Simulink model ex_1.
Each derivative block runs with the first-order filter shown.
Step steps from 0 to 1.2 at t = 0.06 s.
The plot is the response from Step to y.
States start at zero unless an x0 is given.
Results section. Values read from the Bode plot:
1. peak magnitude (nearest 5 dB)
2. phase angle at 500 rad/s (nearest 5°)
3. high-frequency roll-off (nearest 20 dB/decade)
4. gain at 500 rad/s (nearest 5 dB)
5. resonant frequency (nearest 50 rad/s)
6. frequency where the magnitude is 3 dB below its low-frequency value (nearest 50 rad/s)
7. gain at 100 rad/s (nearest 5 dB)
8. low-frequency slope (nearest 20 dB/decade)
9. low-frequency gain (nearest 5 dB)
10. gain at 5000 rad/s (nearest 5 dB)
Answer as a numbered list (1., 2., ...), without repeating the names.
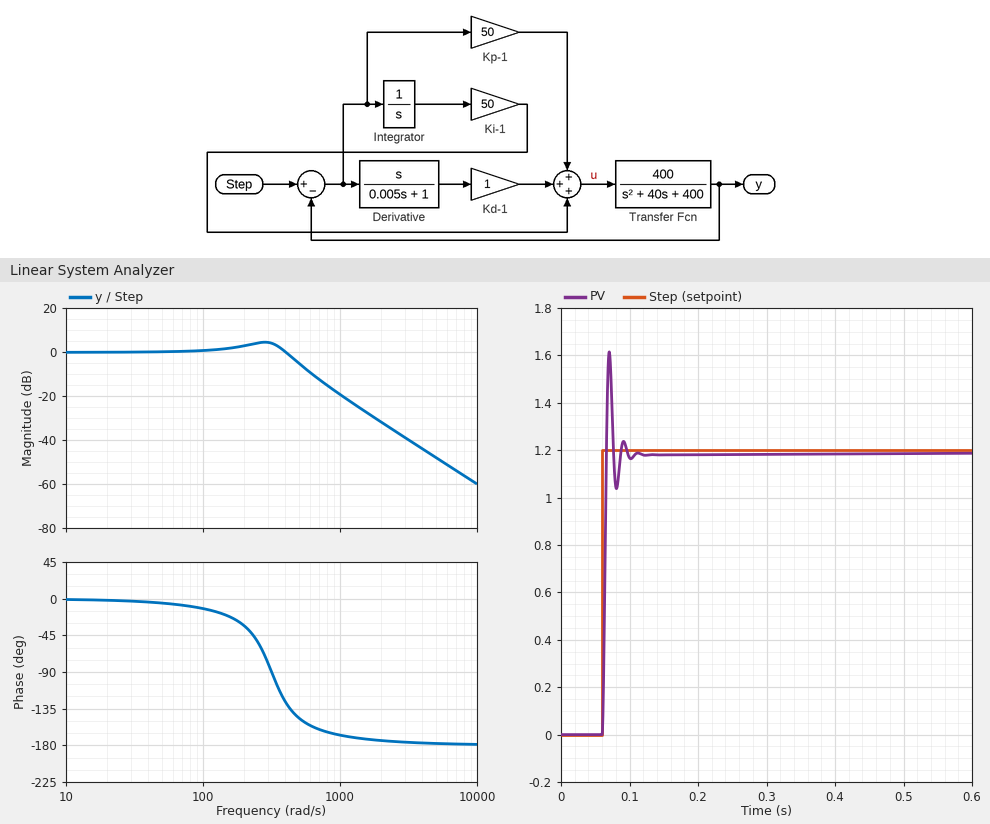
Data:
1. 5 dB
2. -145°
3. -40 dB/decade
4. -5 dB
5. 300 rad/s
6. 450 rad/s
7. 0 dB
8. 0 dB/decade
9. 0 dB
10. -50 dB
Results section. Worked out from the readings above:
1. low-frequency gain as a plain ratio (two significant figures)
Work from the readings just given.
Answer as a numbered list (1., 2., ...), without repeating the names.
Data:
1. 1.0
